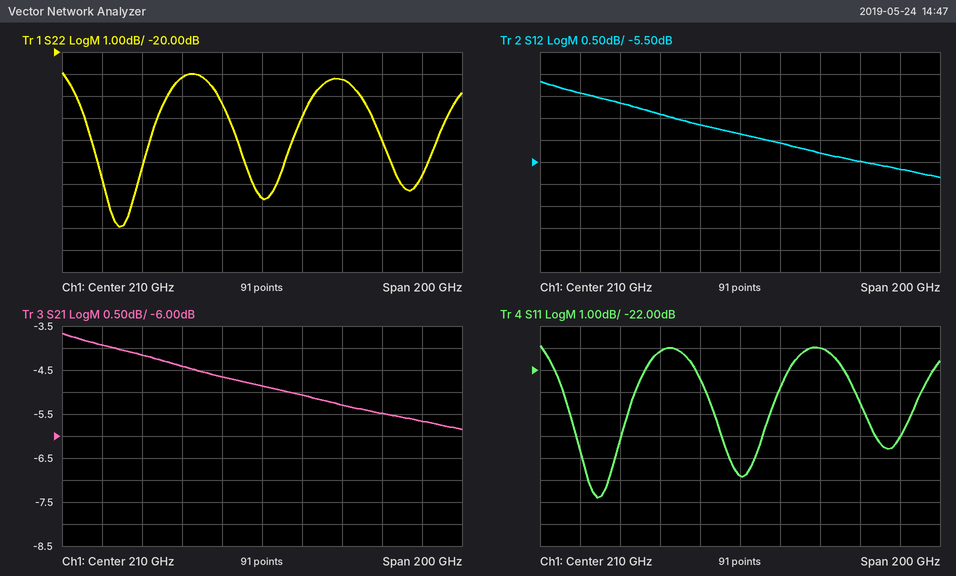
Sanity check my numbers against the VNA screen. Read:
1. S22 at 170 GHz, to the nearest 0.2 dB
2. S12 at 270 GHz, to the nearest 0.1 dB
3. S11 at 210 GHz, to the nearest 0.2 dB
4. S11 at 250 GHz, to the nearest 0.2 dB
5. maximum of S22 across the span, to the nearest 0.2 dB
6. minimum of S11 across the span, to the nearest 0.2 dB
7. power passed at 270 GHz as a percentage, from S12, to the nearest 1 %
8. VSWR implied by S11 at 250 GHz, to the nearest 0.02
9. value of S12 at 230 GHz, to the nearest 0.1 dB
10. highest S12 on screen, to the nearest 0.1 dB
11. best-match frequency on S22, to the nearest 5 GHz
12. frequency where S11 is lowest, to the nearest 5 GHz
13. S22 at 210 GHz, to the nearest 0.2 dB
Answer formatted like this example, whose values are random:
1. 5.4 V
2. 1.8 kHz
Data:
1. -21.2 dB
2. -5.5 dB
3. -26.8 dB
4. -21.0 dB
5. -21.0 dB
6. -27.8 dB
7. 28 %
8. 1.20
9. -5.1 dB
10. -3.7 dB
11. 140 GHz
12. 140 GHz
13. -26.6 dB
